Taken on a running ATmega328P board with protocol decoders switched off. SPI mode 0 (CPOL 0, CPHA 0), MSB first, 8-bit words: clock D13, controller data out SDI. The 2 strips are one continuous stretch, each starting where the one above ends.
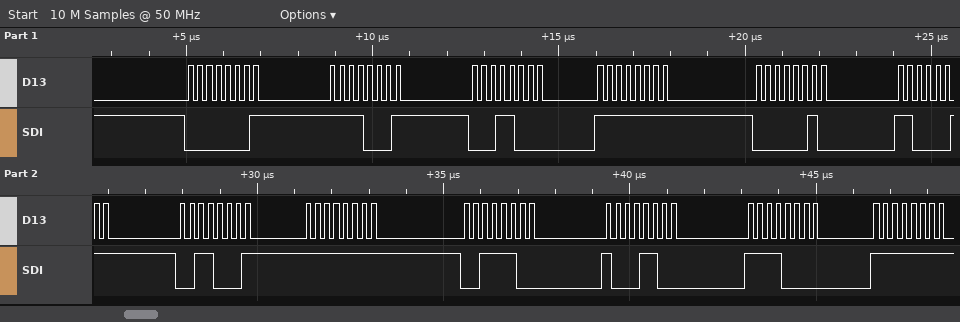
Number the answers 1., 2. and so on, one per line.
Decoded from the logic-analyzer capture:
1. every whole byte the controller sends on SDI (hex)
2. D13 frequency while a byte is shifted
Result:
1. 01 F1 18 FF 02 C3 31 FF 3C 8C F0 FF
2. 4 MHz
